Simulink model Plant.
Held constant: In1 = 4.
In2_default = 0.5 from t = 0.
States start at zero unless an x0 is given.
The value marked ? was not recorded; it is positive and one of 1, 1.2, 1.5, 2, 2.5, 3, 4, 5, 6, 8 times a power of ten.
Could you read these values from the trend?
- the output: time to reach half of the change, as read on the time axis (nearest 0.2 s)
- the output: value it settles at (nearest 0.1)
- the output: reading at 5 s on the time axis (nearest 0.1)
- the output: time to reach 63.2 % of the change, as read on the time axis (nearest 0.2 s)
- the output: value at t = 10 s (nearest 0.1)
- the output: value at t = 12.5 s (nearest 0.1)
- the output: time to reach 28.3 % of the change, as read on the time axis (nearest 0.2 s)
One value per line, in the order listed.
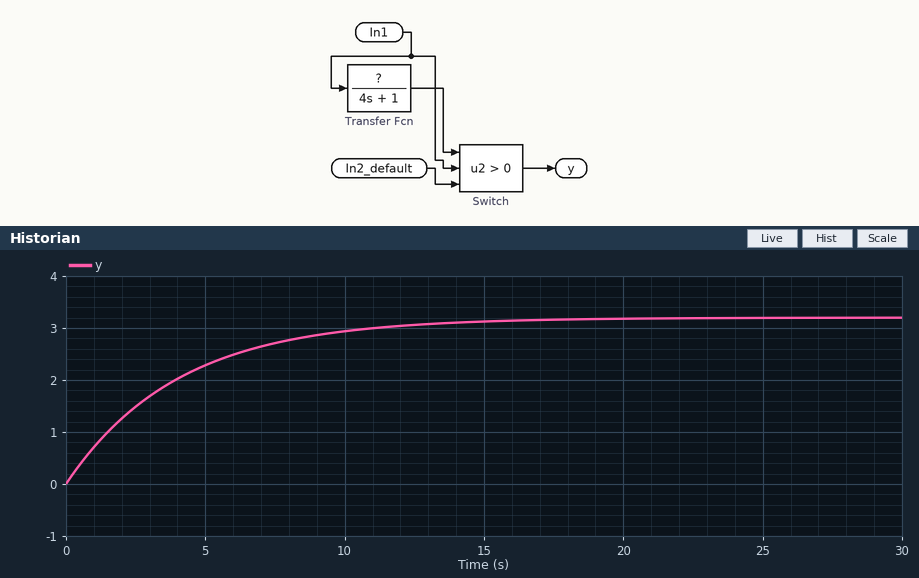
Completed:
2.8 s
3.2
2.3
4.0 s
2.9
3.1
1.4 s
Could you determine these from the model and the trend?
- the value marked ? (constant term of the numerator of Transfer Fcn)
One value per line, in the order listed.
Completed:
0.8
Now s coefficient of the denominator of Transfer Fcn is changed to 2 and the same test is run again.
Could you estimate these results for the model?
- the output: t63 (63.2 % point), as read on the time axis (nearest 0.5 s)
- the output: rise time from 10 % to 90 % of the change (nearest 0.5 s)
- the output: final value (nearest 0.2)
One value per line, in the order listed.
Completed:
2.0 s
4.5 s
3.2
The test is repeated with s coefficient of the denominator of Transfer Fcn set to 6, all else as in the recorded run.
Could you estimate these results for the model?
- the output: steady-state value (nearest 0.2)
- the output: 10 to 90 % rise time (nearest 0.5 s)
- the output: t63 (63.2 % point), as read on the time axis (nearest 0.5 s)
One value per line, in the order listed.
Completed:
3.2
13.0 s
6.0 s
